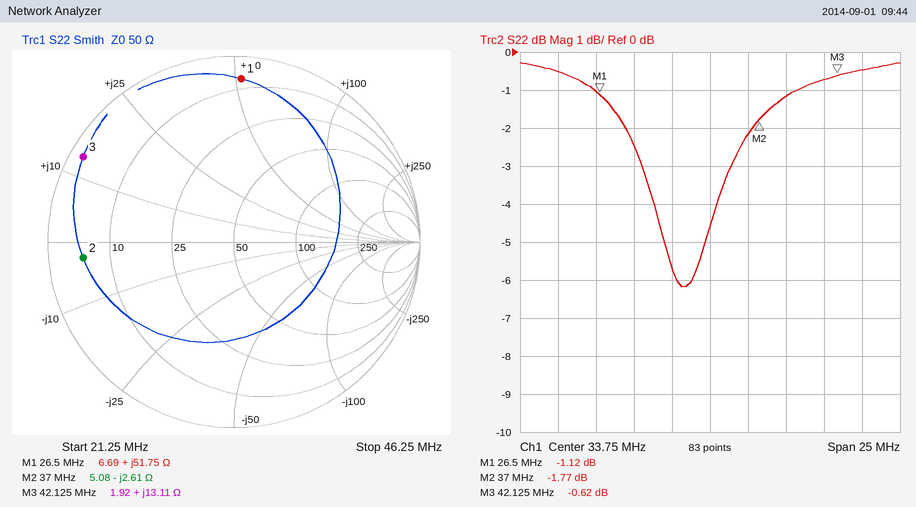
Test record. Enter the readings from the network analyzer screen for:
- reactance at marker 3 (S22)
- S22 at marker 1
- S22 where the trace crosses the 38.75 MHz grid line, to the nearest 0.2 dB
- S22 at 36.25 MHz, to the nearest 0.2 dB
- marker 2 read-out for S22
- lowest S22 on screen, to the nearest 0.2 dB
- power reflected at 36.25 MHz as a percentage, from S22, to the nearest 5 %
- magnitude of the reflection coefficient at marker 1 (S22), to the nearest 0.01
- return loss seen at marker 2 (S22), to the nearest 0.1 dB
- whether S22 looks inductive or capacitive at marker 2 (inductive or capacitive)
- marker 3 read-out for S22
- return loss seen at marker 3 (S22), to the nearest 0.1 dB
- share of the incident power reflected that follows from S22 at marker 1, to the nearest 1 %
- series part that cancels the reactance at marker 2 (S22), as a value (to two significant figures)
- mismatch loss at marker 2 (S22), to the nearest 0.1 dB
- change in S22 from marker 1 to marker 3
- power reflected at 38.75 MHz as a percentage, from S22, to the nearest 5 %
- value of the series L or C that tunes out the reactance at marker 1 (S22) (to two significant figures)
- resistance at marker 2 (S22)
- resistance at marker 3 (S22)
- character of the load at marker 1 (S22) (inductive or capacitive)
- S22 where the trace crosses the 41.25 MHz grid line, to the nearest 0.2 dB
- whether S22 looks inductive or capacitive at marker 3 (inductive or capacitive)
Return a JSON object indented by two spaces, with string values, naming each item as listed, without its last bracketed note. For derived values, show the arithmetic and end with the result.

{
  "reactance at marker 3": "+13.11 Ω",
  "S22 at marker 1": "-1.12 dB",
  "S22 where the trace crosses the 38.75 MHz grid line, to the nearest 0.2 dB": "-1.2 dB",
  "S22 at 36.25 MHz, to the nearest 0.2 dB": "-2.2 dB",
  "marker 2 read-out for S22": "-1.77 dB",
  "lowest S22 on screen, to the nearest 0.2 dB": "-6.2 dB",
  "power reflected at 36.25 MHz as a percentage, from S22, to the nearest 5 %": "10^(-2.2/10) ≈ 60 %",
  "magnitude of the reflection coefficient at marker 1 (S22), to the nearest 0.01": "0.88",
  "return loss seen at marker 2 (S22), to the nearest 0.1 dB": "1.8 dB",
  "whether S22 looks inductive or capacitive at marker 2": "capacitive",
  "marker 3 read-out for S22": "-0.62 dB",
  "return loss seen at marker 3 (S22), to the nearest 0.1 dB": "0.6 dB",
  "share of the incident power reflected that follows from S22 at marker 1, to the nearest 1 %": "10^(-1.12/10) ≈ 77 %",
  "series part that cancels the reactance at marker 2 (S22), as a value": "L = 2.61 Ω/(2π × 37 MHz) ≈ 11 nH",
  "mismatch loss at marker 2 (S22), to the nearest 0.1 dB": "−10 log10(1 − 10^(-1.77/10)) ≈ 4.8 dB",
  "change in S22 from marker 1 to marker 3": "-0.62 − (-1.12) = 0.50 dB",
  "power reflected at 38.75 MHz as a percentage, from S22, to the nearest 5 %": "10^(-1.2/10) ≈ 75.9 %, so 75 % to the nearest 5 %",
  "value of the series L or C that tunes out the reactance at marker 1 (S22)": "C = 1/(2π × 26.5 MHz × 51.75 Ω) ≈ 116 pF, so 120 pF to two significant figures",
  "resistance at marker 2": "5.08 Ω",
  "resistance at marker 3": "1.92 Ω",
  "character of the load at marker 1 (S22)": "inductive",
  "S22 where the trace crosses the 41.25 MHz grid line, to the nearest 0.2 dB": "-0.8 dB",
  "whether S22 looks inductive or capacitive at marker 3": "inductive"
}
